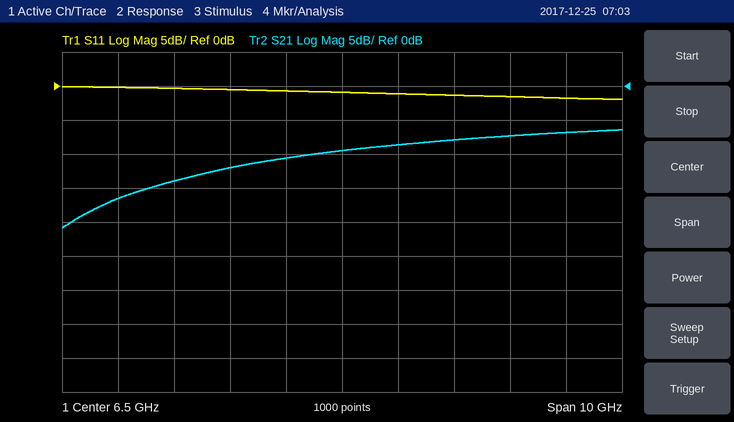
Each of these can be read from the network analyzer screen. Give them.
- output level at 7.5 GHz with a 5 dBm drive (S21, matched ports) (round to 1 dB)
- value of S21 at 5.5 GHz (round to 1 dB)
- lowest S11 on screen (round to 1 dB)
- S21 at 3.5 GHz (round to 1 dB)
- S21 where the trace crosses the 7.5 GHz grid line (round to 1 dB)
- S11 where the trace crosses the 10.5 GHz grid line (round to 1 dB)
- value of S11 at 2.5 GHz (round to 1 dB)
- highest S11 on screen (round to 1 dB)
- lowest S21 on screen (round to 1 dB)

-4 dBm
-11 dB
-2 dB
-14 dB
-9 dB
-2 dB
0 dB
0 dB
-21 dB
